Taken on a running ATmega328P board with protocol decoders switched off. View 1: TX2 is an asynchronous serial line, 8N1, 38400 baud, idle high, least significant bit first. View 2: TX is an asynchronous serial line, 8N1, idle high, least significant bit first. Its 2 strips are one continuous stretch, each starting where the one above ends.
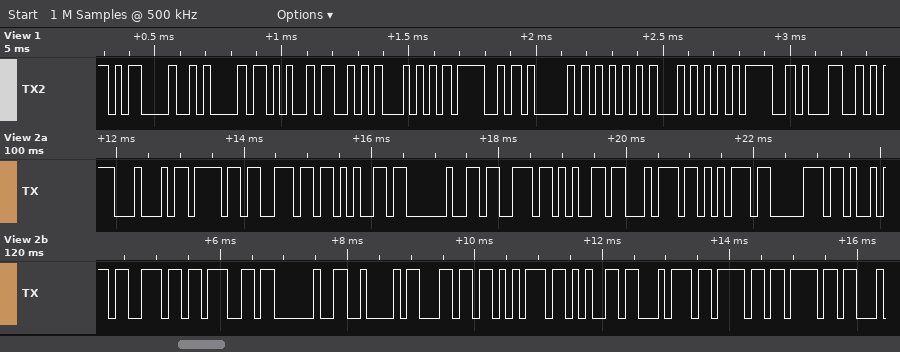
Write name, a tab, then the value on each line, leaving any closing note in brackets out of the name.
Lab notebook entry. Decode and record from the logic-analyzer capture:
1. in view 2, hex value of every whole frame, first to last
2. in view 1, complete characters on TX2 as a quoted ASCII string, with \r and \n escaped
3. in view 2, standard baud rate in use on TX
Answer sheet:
in view 2, hex value of every whole frame, first to last	44 6F 6E 65 20 73 65 74 75 70 69 6E 67 20 42 6C 75 65 74 6F 6F
in view 1, complete characters on TX2 as a quoted ASCII string, with \r and \n escaped	"\r\n+STOAUT=1"
in view 2, standard baud rate in use on TX	9600 baud
